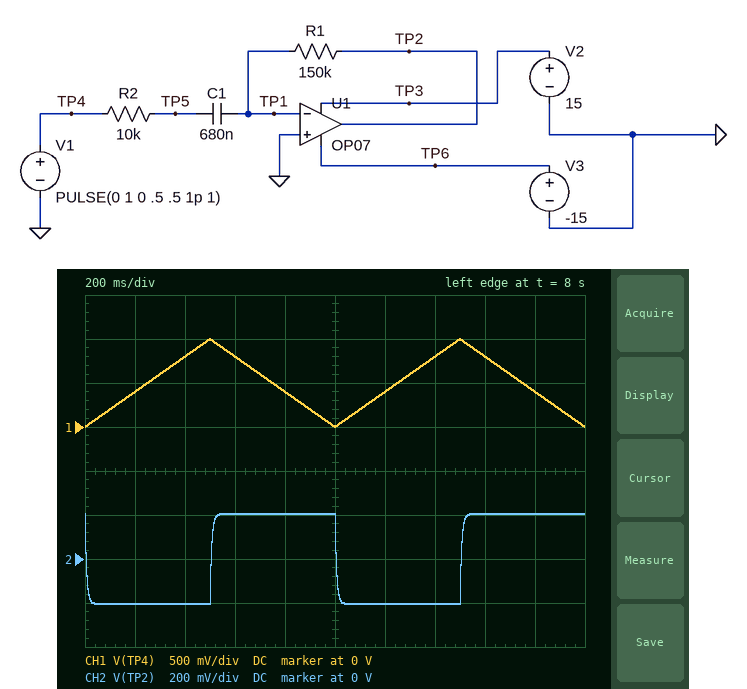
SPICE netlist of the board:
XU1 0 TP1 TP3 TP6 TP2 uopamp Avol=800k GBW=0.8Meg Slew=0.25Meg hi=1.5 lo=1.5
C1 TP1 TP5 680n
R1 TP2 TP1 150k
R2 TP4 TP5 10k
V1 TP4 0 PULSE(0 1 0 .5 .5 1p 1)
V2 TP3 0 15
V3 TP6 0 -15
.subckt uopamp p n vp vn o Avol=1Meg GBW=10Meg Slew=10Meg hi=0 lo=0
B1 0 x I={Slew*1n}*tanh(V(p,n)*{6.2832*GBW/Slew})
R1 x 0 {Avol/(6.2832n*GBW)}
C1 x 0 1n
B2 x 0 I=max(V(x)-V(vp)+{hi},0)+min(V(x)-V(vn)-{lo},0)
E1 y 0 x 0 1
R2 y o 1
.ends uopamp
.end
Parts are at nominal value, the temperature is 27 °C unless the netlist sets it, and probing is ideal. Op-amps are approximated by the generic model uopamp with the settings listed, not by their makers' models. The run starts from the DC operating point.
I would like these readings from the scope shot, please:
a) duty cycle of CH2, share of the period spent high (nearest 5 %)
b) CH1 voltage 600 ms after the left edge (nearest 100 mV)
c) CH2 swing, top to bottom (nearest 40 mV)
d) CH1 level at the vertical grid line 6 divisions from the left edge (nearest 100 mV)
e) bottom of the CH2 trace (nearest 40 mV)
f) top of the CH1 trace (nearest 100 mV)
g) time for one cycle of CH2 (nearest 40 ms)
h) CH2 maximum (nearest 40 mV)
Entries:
50 %
800 mV
400 mV
400 mV
-200 mV
1.0 V
1.00 s
200 mV
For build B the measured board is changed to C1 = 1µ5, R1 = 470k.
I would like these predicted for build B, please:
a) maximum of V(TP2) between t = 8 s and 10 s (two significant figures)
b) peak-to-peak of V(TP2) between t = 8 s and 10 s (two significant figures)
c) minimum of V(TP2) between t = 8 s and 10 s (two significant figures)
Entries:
1.4 V
2.8 V
-1.4 V
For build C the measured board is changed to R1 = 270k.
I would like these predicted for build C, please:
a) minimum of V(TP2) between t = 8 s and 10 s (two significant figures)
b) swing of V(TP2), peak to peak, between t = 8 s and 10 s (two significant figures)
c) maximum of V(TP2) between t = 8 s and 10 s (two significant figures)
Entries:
-370 mV
730 mV
370 mV
